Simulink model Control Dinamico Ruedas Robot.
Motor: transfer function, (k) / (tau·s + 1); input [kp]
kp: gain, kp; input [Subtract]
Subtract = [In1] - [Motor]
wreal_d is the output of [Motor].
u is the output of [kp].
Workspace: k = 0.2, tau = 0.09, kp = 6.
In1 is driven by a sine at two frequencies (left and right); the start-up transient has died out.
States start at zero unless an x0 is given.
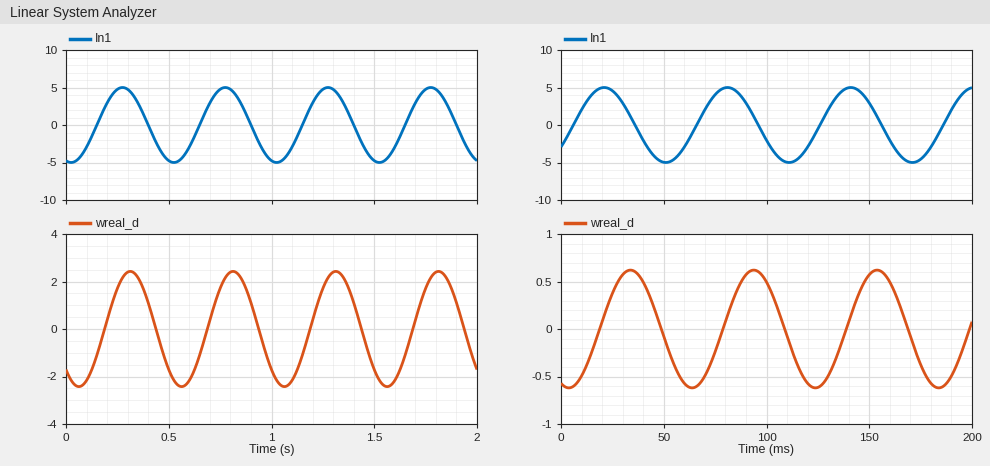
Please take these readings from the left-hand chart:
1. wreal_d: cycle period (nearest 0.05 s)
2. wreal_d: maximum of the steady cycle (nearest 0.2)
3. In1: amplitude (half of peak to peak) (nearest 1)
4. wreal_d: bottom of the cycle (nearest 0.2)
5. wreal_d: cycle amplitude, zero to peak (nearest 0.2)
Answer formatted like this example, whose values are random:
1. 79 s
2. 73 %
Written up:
1. 0.50 s
2. 2.4
3. 5
4. -2.4
5. 2.4
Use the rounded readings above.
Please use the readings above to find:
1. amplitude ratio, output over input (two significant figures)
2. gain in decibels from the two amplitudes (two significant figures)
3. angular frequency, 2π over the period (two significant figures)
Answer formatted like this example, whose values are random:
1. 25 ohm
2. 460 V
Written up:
1. 0.48
2. -6.4 dB
3. 13 rad/s
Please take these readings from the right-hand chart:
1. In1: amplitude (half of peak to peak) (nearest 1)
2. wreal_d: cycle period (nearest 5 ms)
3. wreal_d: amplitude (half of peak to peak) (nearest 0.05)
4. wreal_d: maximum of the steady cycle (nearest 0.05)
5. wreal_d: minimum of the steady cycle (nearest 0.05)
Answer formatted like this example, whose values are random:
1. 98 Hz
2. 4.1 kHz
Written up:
1. 5
2. 60 ms
3. 0.60
4. 0.60
5. -0.60
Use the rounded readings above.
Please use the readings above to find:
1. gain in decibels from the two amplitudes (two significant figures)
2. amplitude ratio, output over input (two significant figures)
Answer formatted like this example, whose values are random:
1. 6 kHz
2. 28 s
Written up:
1. -18 dB
2. 0.12
